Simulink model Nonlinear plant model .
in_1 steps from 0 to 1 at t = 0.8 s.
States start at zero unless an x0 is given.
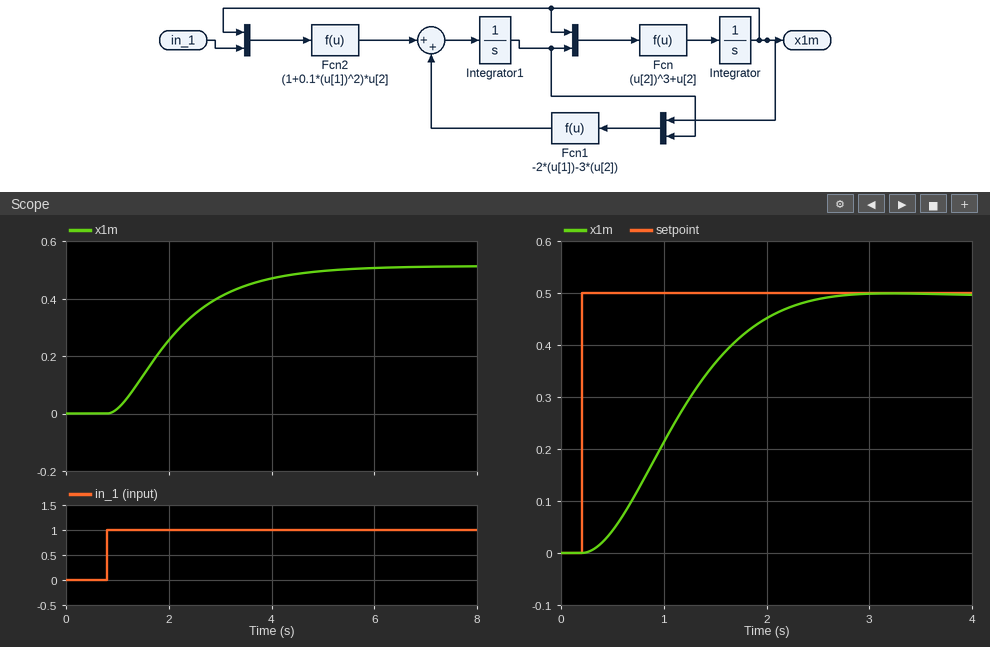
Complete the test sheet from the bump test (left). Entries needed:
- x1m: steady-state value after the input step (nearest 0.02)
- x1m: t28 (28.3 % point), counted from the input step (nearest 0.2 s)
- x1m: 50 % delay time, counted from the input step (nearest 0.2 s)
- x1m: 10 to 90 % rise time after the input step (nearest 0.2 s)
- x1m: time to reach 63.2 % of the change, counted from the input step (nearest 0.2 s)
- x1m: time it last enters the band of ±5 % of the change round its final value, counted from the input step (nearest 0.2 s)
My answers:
0.52
0.8 s
1.2 s
2.6 s
1.6 s
3.8 s
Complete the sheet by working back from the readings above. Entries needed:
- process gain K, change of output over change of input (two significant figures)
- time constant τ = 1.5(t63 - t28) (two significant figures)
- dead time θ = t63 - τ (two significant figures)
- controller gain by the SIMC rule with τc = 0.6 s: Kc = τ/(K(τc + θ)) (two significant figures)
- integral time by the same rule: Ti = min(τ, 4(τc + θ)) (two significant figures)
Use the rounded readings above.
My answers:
0.52
1.2 s
0.40 s
2.3
1.2 s
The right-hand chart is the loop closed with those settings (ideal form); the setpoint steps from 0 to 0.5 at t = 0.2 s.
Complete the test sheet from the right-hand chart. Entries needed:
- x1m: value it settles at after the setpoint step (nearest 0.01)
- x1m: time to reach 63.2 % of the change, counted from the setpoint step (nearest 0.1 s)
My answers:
0.50
1.1 s
